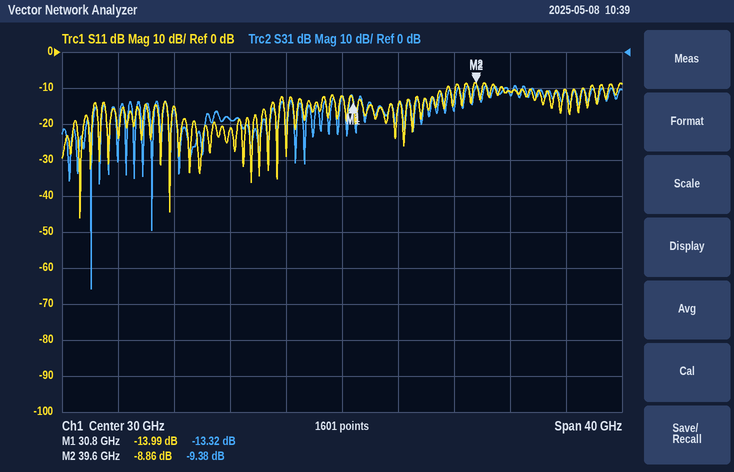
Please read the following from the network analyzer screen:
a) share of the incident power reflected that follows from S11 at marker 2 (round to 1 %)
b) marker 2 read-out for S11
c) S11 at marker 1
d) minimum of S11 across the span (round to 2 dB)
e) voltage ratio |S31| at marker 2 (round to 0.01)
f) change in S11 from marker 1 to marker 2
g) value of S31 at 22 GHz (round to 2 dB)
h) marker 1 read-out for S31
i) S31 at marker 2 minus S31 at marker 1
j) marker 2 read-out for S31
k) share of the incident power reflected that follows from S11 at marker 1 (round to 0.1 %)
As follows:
13 %
-8.86 dB
-13.99 dB
-46 dB
0.34
5.13 dB
-18 dB
-13.32 dB
3.94 dB
-9.38 dB
4.0 %
